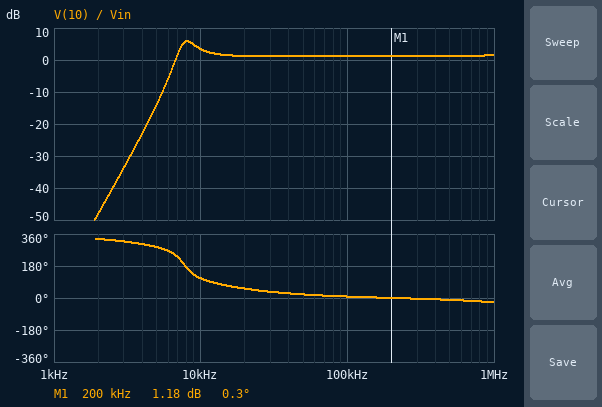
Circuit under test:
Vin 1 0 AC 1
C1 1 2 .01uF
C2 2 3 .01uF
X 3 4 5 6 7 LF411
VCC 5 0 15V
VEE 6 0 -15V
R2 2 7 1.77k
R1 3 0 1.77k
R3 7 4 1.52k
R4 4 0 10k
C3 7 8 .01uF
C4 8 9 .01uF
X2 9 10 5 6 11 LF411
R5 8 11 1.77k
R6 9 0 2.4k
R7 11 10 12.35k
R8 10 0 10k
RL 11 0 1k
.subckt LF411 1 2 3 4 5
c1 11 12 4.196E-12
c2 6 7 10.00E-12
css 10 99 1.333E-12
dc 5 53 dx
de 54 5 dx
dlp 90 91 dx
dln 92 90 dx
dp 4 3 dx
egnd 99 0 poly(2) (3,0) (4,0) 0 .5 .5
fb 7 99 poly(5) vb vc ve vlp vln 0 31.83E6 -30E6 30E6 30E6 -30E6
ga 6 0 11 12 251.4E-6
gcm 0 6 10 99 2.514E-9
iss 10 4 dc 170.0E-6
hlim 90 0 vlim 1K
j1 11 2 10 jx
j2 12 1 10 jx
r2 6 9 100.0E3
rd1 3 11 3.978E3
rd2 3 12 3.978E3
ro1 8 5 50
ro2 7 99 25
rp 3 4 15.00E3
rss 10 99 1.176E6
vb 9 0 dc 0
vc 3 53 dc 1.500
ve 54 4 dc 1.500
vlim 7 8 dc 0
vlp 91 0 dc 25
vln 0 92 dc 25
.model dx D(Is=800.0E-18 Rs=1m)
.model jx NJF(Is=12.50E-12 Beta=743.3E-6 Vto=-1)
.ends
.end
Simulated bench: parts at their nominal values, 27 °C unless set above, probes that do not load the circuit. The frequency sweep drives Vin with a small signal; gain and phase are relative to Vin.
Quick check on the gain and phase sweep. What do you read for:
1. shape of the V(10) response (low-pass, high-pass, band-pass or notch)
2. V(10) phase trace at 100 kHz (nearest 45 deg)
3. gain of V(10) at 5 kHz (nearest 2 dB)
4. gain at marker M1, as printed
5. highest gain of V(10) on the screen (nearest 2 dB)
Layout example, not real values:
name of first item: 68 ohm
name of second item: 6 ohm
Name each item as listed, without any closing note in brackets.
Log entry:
shape of the V(10) response: high-pass
V(10) phase trace at 100 kHz: 0 deg
gain of V(10) at 5 kHz: -14 dB
gain at marker M1, as printed: 1.18 dB
highest gain of V(10) on the screen: 6 dB
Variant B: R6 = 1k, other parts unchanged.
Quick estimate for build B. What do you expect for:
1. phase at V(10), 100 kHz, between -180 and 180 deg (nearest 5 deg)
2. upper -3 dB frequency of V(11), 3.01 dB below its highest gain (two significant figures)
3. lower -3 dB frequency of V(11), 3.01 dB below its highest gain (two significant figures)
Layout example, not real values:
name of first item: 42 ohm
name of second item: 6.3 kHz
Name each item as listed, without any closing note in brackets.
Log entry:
phase at V(10), 100 kHz, between -180 and 180 deg: 20 deg
upper -3 dB frequency of V(11), 3.01 dB below its highest gain: 4.7 MHz
lower -3 dB frequency of V(11), 3.01 dB below its highest gain: 29 kHz
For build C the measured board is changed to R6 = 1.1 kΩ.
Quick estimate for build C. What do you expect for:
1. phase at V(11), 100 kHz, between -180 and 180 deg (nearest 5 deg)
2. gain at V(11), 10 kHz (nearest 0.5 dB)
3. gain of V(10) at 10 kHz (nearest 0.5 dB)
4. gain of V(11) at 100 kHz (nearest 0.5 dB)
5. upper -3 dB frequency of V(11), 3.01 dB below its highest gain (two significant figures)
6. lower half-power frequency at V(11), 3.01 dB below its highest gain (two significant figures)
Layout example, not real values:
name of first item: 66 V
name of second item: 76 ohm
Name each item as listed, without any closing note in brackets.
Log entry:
phase at V(11), 100 kHz, between -180 and 180 deg: 15 deg
gain at V(11), 10 kHz: -1.5 dB
gain of V(10) at 10 kHz: -8.5 dB
gain of V(11) at 100 kHz: 8.0 dB
upper -3 dB frequency of V(11), 3.01 dB below its highest gain: 4.7 MHz
lower half-power frequency at V(11), 3.01 dB below its highest gain: 24 kHz
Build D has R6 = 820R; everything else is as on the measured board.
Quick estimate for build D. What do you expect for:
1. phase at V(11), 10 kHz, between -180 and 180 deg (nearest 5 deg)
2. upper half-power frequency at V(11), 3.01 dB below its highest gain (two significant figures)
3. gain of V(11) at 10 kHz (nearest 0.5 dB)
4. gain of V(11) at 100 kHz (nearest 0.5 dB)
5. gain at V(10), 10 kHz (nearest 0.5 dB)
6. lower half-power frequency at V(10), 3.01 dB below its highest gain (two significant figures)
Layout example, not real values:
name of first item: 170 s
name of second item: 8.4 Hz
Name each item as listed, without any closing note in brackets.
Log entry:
phase at V(11), 10 kHz, between -180 and 180 deg: -170 deg
upper half-power frequency at V(11), 3.01 dB below its highest gain: 4.7 MHz
gain of V(11) at 10 kHz: -5.5 dB
gain of V(11) at 100 kHz: 8.0 dB
gain at V(10), 10 kHz: -12.5 dB
lower half-power frequency at V(10), 3.01 dB below its highest gain: 39 kHz
